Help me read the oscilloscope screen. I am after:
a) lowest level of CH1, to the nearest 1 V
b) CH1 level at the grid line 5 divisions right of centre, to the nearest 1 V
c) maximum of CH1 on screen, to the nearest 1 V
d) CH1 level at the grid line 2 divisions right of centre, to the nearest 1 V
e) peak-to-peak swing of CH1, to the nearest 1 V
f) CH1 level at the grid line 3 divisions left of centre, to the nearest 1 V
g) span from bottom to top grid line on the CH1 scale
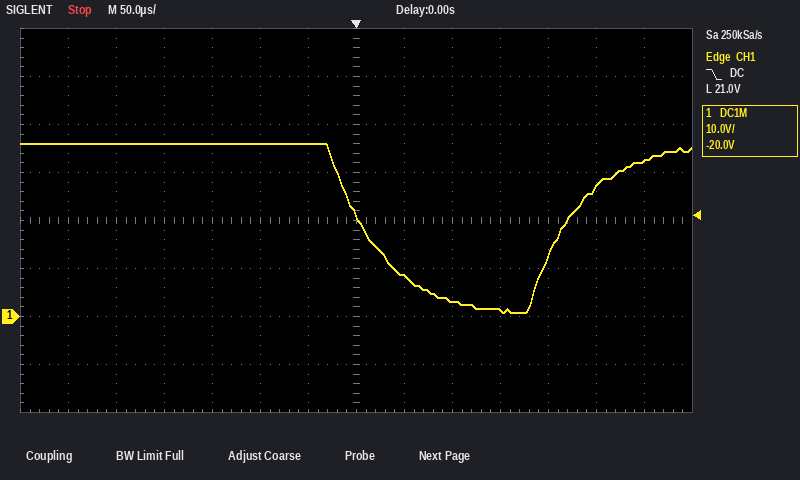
1 V
27 V
36 V
3 V
35 V
36 V
80 V
